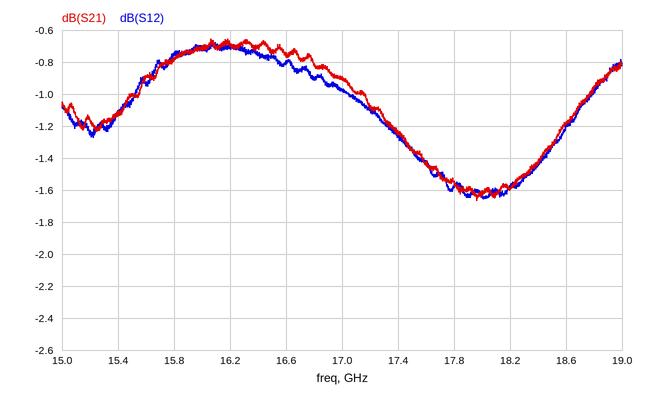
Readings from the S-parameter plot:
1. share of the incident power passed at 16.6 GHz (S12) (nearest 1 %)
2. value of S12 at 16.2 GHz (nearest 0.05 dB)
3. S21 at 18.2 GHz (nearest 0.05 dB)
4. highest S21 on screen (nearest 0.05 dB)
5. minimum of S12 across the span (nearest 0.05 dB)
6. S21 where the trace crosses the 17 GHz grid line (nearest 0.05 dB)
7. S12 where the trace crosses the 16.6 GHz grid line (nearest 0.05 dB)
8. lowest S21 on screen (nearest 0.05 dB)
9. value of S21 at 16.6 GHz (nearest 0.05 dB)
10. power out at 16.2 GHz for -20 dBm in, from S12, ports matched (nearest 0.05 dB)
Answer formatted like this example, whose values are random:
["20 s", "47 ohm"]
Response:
["83 %", "-0.70 dB", "-1.60 dB", "-0.65 dB", "-1.65 dB", "-0.90 dB", "-0.80 dB", "-1.65 dB", "-0.75 dB", "-20.70 dBm"]
